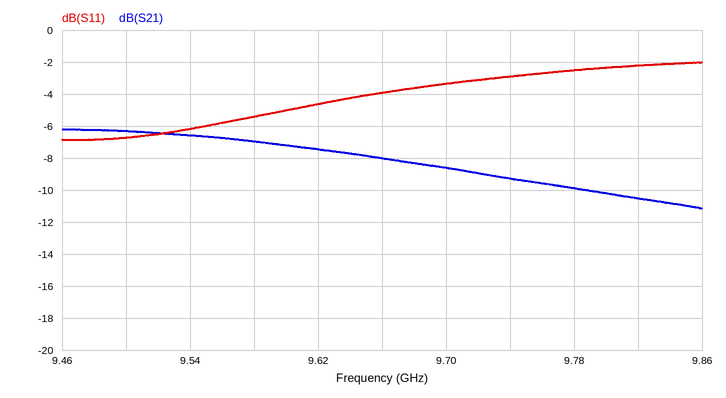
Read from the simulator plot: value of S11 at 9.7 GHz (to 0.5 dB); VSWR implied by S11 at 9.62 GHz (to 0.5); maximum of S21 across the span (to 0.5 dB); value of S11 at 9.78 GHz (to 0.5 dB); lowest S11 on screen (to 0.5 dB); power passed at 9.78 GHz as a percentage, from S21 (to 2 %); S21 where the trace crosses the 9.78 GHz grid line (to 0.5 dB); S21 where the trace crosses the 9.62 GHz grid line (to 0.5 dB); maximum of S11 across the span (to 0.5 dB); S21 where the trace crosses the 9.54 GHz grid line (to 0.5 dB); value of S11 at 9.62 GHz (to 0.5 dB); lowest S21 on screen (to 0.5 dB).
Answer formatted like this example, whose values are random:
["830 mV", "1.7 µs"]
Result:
["-3.5 dB", "4.0", "-6.0 dB", "-2.5 dB", "-7.0 dB", "10 %", "-10.0 dB", "-7.5 dB", "-2.0 dB", "-6.5 dB", "-4.5 dB", "-11.0 dB"]
